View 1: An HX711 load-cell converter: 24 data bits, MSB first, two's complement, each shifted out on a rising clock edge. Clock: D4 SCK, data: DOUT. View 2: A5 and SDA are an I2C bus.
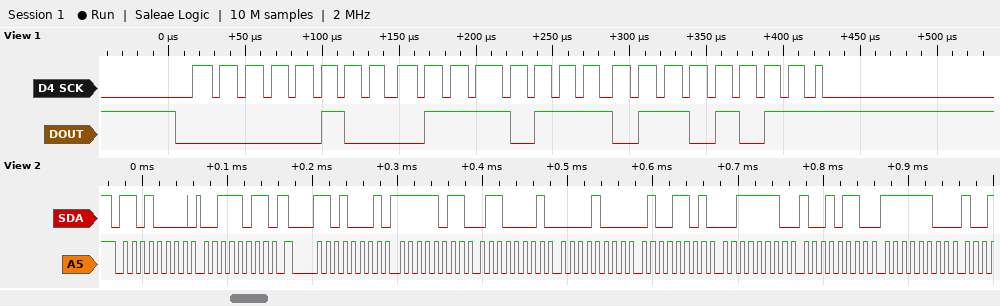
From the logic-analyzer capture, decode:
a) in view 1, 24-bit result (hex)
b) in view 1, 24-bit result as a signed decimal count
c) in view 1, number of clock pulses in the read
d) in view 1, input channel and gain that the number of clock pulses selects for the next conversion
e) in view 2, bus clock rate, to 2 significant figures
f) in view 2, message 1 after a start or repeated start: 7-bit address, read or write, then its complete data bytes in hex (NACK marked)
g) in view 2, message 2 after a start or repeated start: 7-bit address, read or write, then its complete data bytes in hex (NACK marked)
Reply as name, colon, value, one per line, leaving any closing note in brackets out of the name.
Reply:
in view 1, 24-bit result: 0x04776B
in view 1, 24-bit result as a signed decimal count: 292715
in view 1, number of clock pulses in the read: 25
in view 1, input channel and gain that the number of clock pulses selects for the next conversion: channel A, gain 128
in view 2, bus clock rate, to 2 significant figures: 100 kHz
in view 2, message 1 after a start or repeated start: 7-bit address, read or write, then its complete data bytes in hex: 0x68 write: 3B
in view 2, message 2 after a start or repeated start: 7-bit address, read or write, then its complete data bytes in hex: 0x68 read: FB 61 08 4D 3E 96 FC
